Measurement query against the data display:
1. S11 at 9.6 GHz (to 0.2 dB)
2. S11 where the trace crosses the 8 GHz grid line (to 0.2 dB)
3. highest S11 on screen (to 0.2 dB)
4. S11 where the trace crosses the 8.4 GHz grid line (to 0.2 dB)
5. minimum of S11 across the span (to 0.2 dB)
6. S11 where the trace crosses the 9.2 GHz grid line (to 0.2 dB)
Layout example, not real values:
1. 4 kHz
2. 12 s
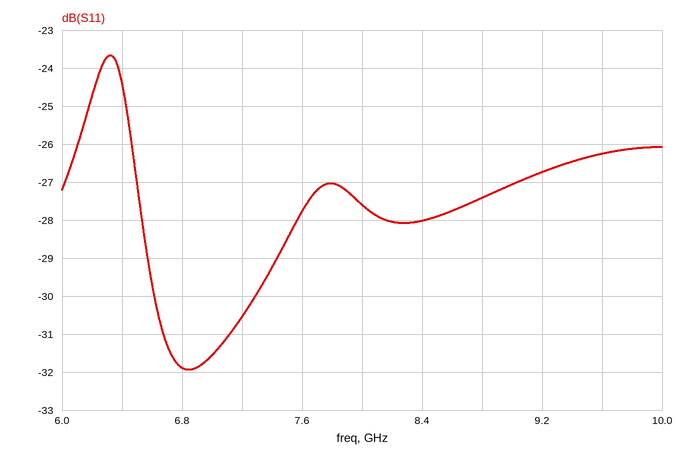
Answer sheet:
1. -26.2 dB
2. -27.6 dB
3. -23.6 dB
4. -28.0 dB
5. -32.0 dB
6. -26.8 dB
